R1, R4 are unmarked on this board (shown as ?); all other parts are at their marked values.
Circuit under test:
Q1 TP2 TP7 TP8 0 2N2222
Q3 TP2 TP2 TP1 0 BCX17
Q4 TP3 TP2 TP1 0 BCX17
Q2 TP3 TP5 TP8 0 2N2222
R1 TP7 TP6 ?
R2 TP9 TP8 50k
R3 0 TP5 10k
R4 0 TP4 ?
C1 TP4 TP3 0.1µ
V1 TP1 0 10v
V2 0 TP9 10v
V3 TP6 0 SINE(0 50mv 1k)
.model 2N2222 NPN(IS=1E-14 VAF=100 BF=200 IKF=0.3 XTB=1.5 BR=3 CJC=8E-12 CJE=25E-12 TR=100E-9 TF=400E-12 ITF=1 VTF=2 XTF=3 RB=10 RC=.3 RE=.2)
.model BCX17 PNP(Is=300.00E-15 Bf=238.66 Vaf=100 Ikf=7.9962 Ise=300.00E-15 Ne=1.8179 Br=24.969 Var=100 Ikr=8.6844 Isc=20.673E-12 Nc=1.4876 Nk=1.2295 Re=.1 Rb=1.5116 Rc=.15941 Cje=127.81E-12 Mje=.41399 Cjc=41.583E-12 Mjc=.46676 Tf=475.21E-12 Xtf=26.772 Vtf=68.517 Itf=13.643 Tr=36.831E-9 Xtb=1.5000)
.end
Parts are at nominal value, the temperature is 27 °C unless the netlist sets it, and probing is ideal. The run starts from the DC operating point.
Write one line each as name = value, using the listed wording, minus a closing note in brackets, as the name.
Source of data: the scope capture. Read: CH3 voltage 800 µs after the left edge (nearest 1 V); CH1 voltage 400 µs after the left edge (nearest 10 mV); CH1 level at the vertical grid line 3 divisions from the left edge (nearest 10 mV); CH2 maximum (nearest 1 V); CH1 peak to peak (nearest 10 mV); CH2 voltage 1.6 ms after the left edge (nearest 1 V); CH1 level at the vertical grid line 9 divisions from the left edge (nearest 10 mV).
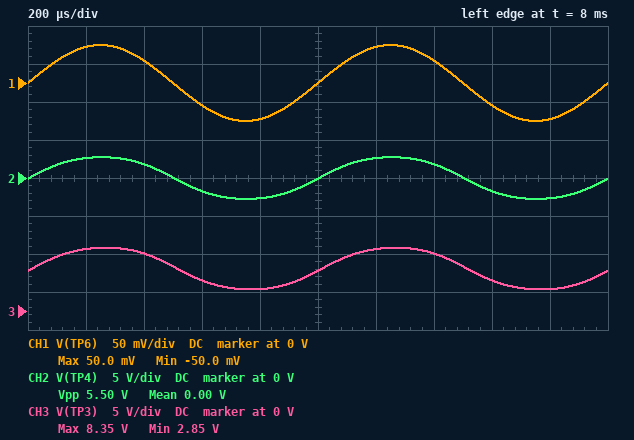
CH3 voltage 800 µs after the left edge = 3 V
CH1 voltage 400 µs after the left edge = 30 mV
CH1 level at the vertical grid line 3 divisions from the left edge = -30 mV
CH2 maximum = 3 V
CH1 peak to peak = 100 mV
CH2 voltage 1.6 ms after the left edge = -2 V
CH1 level at the vertical grid line 9 divisions from the left edge = -50 mV
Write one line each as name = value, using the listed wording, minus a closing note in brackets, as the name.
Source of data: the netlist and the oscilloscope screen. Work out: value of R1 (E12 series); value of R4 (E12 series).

value of R1 = 15 kΩ
value of R4 = 22 kΩ
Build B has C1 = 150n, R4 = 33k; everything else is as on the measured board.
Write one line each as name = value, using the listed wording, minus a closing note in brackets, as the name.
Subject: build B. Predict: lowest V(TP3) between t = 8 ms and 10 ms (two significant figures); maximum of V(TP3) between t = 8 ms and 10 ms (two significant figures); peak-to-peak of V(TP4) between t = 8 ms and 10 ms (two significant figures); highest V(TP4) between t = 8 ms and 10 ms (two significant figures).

lowest V(TP3) between t = 8 ms and 10 ms = 1.4 V
maximum of V(TP3) between t = 8 ms and 10 ms = 9.5 V
peak-to-peak of V(TP4) between t = 8 ms and 10 ms = 8.1 V
highest V(TP4) between t = 8 ms and 10 ms = 4.0 V
